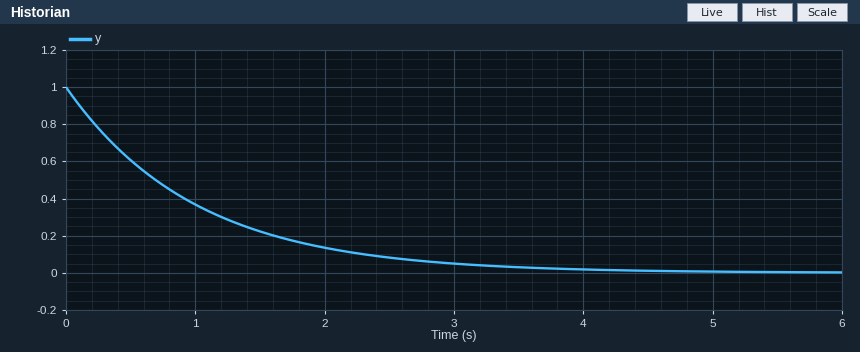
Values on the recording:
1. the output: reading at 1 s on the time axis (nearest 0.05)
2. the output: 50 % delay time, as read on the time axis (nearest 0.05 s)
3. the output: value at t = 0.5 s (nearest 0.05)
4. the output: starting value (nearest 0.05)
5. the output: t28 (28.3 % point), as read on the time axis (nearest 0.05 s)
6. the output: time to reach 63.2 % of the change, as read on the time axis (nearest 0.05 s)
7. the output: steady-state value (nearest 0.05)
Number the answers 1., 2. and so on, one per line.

1. 0.35
2. 0.70 s
3. 0.60
4. 1.00
5. 0.35 s
6. 1.00 s
7. 0.00
